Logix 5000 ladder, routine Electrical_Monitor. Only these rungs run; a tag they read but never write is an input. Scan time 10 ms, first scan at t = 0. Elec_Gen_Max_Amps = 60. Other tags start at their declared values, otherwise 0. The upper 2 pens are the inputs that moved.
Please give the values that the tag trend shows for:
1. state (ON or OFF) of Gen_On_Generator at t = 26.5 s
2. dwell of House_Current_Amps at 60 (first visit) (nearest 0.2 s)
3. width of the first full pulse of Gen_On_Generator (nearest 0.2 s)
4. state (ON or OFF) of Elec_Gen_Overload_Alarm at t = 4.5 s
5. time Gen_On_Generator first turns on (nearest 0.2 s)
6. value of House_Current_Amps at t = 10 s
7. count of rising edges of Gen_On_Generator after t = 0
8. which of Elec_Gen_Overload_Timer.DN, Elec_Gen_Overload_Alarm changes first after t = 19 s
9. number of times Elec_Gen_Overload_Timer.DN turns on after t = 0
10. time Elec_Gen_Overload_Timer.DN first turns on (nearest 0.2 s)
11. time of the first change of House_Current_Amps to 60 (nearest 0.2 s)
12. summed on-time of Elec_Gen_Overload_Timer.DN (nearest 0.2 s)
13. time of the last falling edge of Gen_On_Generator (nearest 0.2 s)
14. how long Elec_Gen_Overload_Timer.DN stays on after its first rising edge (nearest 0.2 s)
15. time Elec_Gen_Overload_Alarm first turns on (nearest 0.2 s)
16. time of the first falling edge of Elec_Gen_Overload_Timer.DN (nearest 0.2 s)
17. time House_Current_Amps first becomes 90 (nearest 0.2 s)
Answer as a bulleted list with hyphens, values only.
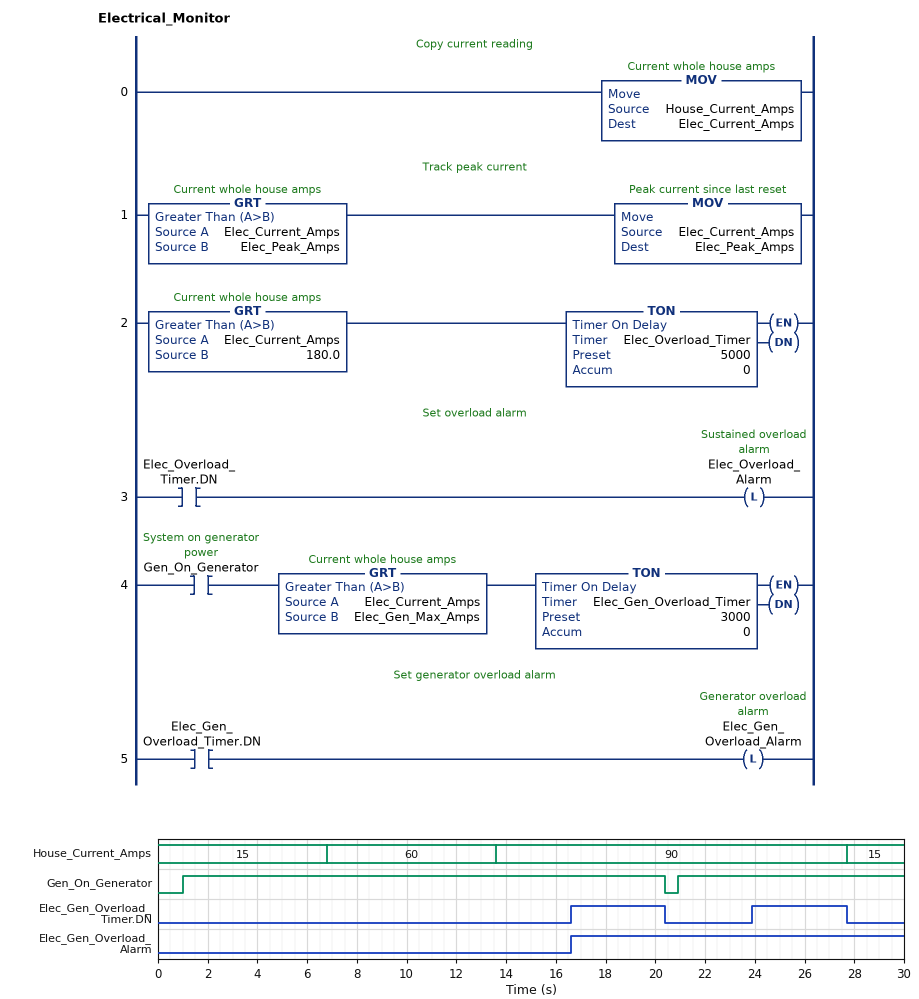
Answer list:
- ON
- 6.8 s
- 19.4 s
- OFF
- 1.0 s
- 60
- 2
- Elec_Gen_Overload_Timer.DN
- 2
- 16.6 s
- 6.8 s
- 7.6 s
- 20.4 s
- 3.8 s
- 16.6 s
- 20.4 s
- 13.6 s
